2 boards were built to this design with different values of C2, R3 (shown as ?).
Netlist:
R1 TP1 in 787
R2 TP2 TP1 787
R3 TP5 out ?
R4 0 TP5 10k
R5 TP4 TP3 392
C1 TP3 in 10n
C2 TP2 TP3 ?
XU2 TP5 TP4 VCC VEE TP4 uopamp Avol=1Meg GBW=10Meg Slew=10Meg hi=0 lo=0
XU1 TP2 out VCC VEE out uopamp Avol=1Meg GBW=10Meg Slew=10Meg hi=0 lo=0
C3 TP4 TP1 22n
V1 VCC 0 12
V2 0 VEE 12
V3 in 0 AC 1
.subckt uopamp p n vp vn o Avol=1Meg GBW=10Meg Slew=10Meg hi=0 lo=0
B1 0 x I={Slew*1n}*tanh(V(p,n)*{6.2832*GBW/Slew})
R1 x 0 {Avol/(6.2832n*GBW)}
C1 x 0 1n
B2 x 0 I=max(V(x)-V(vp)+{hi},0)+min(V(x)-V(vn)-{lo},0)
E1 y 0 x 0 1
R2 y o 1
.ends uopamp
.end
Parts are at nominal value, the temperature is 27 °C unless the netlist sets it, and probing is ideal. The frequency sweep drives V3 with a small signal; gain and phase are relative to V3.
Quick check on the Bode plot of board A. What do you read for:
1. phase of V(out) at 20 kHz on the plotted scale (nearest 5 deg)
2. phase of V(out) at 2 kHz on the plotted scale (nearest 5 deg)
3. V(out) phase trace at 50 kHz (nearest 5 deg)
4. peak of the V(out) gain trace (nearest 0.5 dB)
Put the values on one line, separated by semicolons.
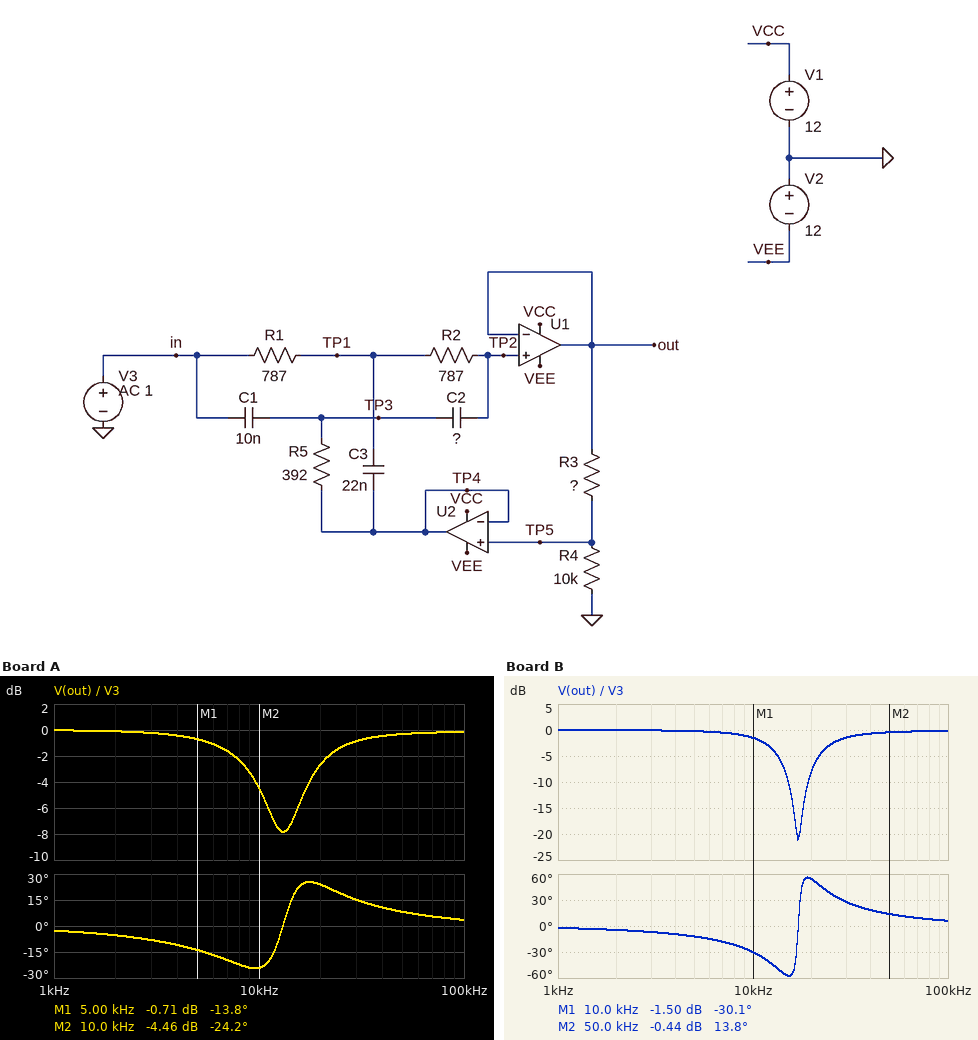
25 deg; -5 deg; 10 deg; 0 dB
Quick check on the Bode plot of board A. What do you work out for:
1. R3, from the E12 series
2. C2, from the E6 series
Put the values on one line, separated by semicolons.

1.2 kΩ; 33 nF
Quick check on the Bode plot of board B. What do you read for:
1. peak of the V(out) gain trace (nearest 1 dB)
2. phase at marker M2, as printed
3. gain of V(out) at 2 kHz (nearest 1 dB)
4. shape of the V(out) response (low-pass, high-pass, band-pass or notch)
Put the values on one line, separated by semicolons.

0 dB; 13.8 deg; 0 dB; notch
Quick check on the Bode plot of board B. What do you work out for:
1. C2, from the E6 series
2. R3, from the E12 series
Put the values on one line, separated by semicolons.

15 nF; 1.8 kΩ
